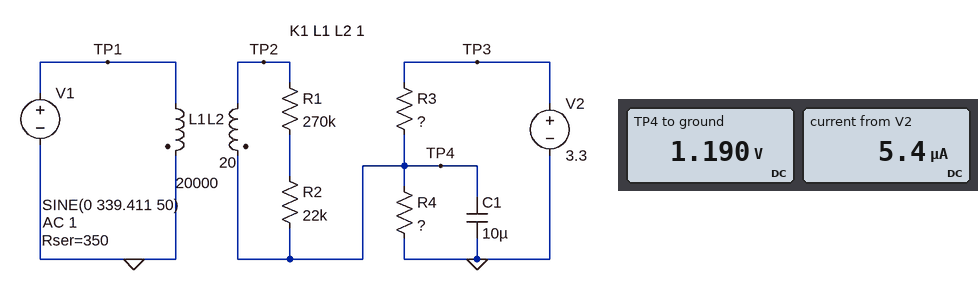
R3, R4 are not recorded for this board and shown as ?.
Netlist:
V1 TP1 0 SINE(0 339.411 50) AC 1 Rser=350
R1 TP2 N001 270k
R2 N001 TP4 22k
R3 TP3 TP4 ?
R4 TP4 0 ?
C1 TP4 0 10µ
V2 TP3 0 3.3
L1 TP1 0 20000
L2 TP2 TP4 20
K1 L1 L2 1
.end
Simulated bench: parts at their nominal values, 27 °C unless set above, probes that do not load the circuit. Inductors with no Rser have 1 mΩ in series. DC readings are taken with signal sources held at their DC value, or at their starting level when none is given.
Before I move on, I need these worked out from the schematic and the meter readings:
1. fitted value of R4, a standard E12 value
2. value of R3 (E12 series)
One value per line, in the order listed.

220 kΩ
390 kΩ
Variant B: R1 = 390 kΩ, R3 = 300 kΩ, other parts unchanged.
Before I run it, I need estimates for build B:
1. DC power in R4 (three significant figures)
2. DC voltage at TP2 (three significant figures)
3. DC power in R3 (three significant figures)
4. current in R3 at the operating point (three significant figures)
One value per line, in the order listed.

8.86 µW
1.40 V
12.1 µW
6.35 µA
